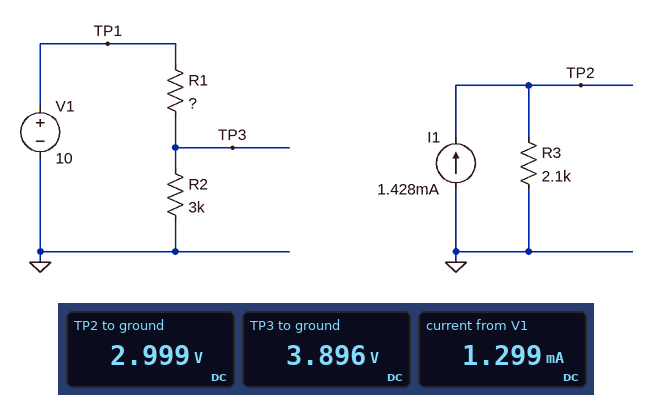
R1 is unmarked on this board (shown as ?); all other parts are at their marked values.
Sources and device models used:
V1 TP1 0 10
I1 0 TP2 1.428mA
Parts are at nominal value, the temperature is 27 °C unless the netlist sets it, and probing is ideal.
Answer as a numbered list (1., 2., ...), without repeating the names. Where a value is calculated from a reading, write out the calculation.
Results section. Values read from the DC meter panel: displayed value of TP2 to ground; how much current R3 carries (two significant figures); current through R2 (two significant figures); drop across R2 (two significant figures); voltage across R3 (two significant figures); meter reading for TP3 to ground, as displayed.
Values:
1. 2.999 V
2. (2.999 V) / 2.1 kΩ = 1.4 mA
3. (3.896 V) / 3 kΩ = 1.3 mA
4. 3.896 V = 3.9 V
5. 2.999 V = 3.0 V
6. 3.896 V
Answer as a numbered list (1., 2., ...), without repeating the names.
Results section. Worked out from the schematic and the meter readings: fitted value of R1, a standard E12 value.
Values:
1. 4.7 kΩ
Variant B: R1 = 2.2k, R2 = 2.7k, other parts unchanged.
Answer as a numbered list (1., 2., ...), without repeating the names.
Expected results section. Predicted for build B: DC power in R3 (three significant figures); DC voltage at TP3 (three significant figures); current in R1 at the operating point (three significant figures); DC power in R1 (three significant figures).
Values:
1. 4.28 mW
2. 5.51 V
3. 2.04 mA
4. 9.16 mW
